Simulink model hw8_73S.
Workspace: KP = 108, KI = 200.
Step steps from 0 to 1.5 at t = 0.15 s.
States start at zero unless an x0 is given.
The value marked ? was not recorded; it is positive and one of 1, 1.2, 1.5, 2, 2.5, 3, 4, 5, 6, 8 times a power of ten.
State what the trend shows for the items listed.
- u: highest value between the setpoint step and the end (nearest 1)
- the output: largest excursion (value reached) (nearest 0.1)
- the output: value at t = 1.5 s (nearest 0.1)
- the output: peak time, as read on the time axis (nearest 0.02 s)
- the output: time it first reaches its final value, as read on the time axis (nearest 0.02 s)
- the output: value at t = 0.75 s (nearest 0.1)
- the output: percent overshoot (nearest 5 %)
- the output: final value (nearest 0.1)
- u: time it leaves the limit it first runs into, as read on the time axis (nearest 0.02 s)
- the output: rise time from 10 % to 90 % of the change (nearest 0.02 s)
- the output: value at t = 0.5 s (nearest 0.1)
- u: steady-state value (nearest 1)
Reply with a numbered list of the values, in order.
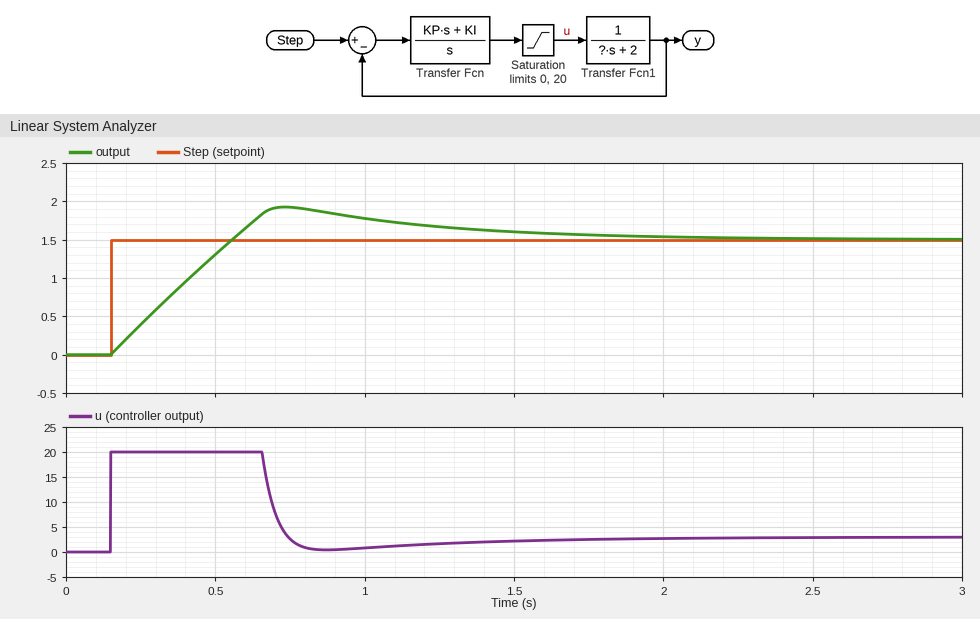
1. 20
2. 1.9
3. 1.6
4. 0.74 s
5. 0.56 s
6. 1.9
7. 30 %
8. 1.5
9. 0.66 s
10. 0.32 s
11. 1.3
12. 3
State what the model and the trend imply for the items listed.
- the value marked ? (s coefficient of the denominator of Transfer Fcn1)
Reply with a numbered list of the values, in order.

1. 5
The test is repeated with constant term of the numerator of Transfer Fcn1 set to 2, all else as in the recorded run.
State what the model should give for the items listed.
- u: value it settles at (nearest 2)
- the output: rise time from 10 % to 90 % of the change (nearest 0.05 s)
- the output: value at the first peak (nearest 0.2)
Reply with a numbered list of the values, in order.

1. 2
2. 0.15 s
3. 1.8
